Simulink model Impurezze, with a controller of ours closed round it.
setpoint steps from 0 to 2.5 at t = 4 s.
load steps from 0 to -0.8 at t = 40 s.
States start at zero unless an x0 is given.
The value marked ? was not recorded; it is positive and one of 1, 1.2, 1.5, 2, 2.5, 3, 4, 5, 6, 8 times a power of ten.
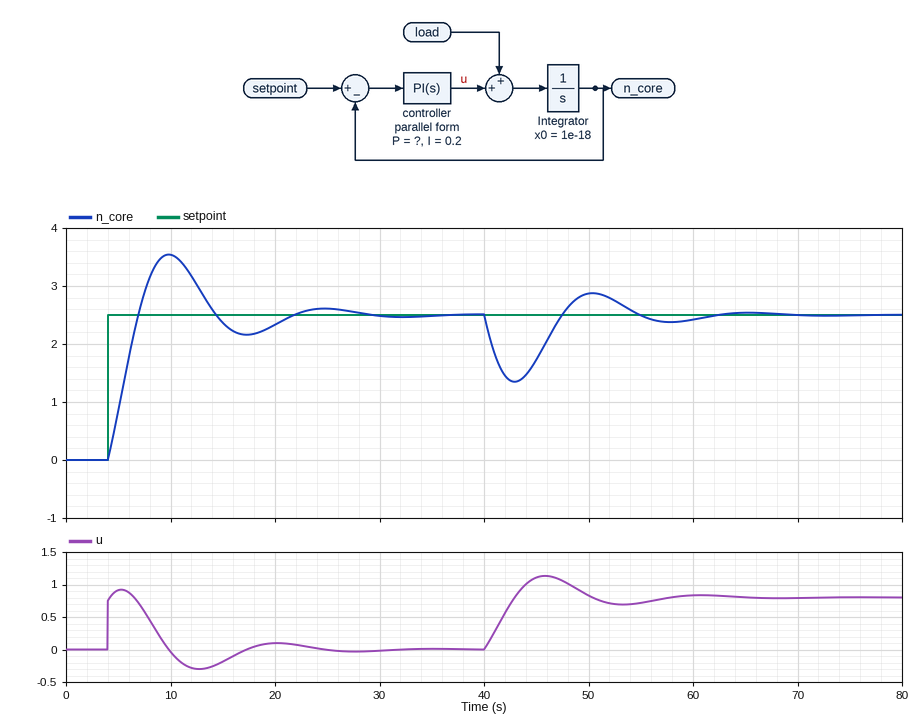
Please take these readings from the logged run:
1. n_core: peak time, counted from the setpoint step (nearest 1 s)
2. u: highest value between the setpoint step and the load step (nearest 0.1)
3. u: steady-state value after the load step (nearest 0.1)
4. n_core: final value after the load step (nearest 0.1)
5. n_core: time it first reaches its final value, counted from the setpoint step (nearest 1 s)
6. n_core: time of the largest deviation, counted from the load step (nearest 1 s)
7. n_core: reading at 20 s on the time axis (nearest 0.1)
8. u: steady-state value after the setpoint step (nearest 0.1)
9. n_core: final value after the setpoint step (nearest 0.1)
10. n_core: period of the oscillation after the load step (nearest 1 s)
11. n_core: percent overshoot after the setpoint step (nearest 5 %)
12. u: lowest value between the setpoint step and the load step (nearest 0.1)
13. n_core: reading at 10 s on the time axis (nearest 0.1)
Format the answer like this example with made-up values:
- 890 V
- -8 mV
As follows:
- 6 s
- 0.9
- 0.8
- 2.5
- 3 s
- 3 s
- 2.3
- 0.0
- 2.5
- 15 s
- 40 %
- -0.3
- 3.5
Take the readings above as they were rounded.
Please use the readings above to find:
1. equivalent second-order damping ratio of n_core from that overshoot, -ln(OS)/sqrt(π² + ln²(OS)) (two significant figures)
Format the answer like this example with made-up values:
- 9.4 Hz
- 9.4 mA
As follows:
- 0.28
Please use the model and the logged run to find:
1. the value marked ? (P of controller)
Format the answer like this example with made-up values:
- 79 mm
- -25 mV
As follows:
- 0.3
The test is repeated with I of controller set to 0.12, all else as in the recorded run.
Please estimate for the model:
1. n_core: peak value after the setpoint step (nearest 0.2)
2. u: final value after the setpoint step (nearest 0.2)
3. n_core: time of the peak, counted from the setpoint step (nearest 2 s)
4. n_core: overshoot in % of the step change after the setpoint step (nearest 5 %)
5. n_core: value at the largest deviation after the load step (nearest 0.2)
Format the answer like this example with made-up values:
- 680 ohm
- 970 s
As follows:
- 3.4
- 0.0
- 8 s
- 35 %
- 1.2
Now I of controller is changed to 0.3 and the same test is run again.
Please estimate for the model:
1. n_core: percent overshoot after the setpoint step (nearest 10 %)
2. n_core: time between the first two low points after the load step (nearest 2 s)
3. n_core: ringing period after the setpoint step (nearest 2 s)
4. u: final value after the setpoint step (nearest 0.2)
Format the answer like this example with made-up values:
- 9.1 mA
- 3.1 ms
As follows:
- 50 %
- 12 s
- 12 s
- 0.0
